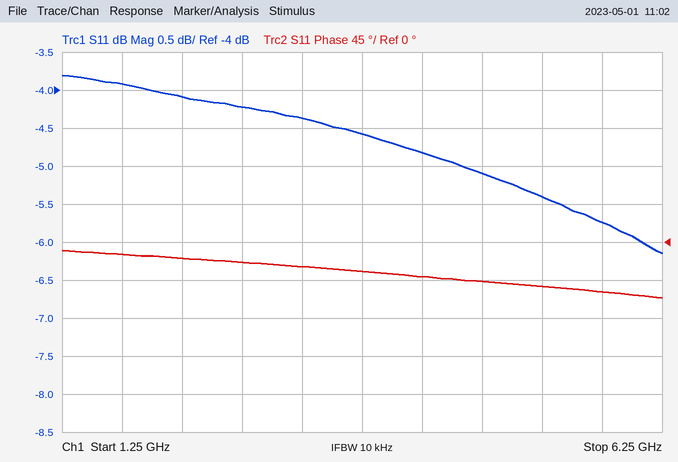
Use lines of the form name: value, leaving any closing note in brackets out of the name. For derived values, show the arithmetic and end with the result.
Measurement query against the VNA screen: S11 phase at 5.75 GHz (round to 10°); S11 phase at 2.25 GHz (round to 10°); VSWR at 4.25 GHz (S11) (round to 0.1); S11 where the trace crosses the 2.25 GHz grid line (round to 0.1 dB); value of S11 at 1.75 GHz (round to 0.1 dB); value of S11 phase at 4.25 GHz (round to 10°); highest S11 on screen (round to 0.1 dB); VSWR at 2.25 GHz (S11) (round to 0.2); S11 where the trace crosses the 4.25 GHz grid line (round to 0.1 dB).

S11 phase at 5.75 GHz: -60°
S11 phase at 2.25 GHz: -20°
VSWR at 4.25 GHz (S11): |Γ| = 10^(-4.8/20) = 0.5754; VSWR = (1 + 0.5754)/(1 − 0.5754) ≈ 3.7
S11 where the trace crosses the 2.25 GHz grid line: -4.1 dB
value of S11 at 1.75 GHz: -3.9 dB
value of S11 phase at 4.25 GHz: -40°
highest S11 on screen: -3.8 dB
VSWR at 2.25 GHz (S11): |Γ| = 10^(-4.1/20) = 0.6237; VSWR = (1 + 0.6237)/(1 − 0.6237) ≈ 4.32, so 4.4 to the nearest 0.2
S11 where the trace crosses the 4.25 GHz grid line: -4.8 dB
